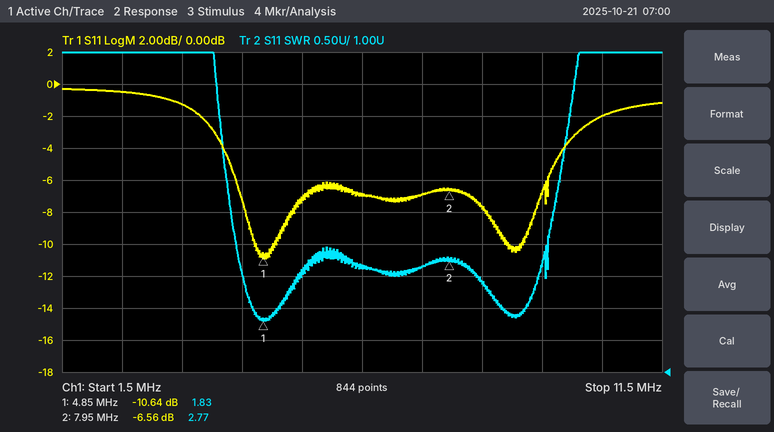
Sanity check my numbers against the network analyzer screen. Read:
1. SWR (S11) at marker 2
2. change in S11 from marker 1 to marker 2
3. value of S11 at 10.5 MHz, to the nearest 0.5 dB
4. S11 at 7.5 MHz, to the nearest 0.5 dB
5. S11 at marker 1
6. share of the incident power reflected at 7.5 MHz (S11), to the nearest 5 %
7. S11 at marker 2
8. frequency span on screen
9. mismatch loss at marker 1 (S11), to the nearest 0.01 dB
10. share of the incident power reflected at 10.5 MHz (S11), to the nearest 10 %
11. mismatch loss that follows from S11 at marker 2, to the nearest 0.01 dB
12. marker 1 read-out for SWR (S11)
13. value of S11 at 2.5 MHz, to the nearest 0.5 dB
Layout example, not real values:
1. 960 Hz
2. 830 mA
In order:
1. 2.77
2. 4.08 dB
3. -2.0 dB
4. -7.0 dB
5. -10.64 dB
6. 20 %
7. -6.56 dB
8. 10 MHz
9. 0.39 dB
10. 60 %
11. 1.08 dB
12. 1.83
13. -0.5 dB
